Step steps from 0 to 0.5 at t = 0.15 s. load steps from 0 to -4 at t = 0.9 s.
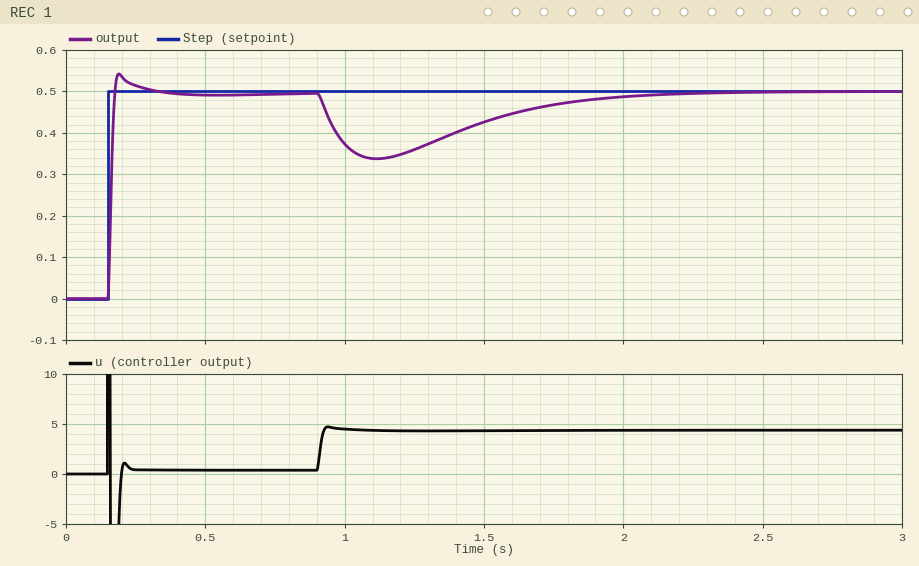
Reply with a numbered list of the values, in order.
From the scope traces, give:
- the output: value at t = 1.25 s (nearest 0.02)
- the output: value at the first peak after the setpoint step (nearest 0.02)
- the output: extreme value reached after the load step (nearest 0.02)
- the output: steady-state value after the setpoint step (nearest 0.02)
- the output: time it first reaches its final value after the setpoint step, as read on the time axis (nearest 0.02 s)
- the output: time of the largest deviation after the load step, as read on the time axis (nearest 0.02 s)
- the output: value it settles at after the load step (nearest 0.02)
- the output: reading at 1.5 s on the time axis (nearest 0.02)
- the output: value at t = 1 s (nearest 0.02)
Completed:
1. 0.36
2. 0.54
3. 0.34
4. 0.50
5. 0.18 s
6. 1.12 s
7. 0.50
8. 0.42
9. 0.38
